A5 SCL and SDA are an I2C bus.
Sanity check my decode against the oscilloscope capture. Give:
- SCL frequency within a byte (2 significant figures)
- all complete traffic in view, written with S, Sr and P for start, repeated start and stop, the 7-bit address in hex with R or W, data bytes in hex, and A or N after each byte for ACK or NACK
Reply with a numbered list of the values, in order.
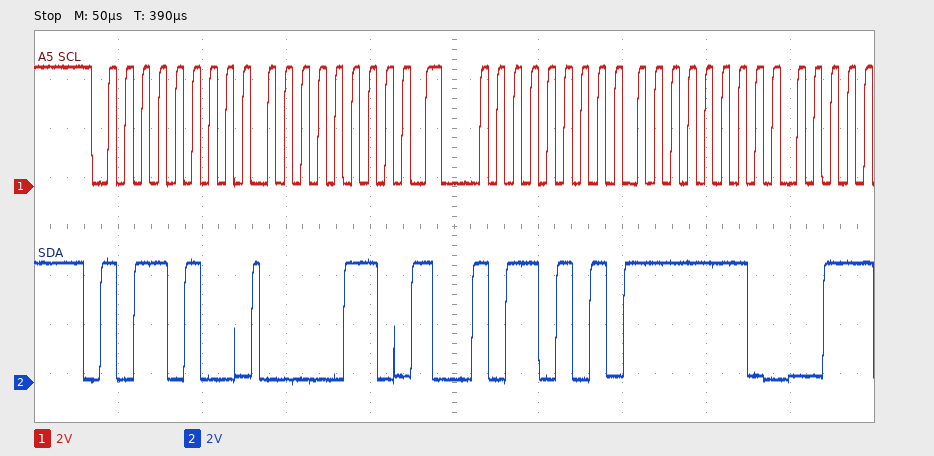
1. 100 kHz
2. S 5AW A 06 A Sr 5AR A FE A
